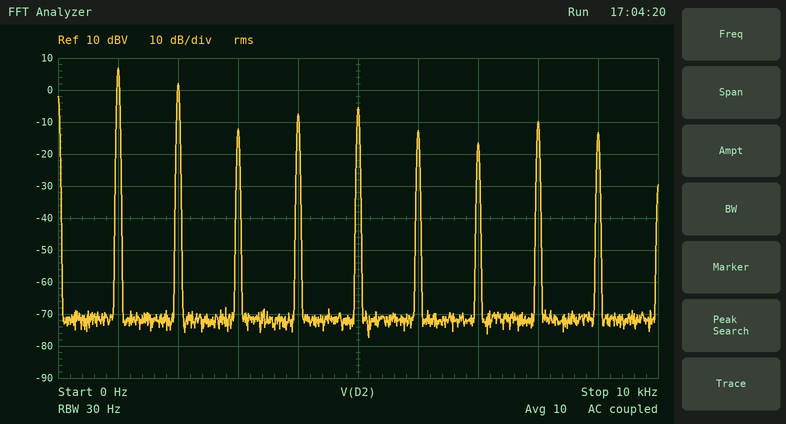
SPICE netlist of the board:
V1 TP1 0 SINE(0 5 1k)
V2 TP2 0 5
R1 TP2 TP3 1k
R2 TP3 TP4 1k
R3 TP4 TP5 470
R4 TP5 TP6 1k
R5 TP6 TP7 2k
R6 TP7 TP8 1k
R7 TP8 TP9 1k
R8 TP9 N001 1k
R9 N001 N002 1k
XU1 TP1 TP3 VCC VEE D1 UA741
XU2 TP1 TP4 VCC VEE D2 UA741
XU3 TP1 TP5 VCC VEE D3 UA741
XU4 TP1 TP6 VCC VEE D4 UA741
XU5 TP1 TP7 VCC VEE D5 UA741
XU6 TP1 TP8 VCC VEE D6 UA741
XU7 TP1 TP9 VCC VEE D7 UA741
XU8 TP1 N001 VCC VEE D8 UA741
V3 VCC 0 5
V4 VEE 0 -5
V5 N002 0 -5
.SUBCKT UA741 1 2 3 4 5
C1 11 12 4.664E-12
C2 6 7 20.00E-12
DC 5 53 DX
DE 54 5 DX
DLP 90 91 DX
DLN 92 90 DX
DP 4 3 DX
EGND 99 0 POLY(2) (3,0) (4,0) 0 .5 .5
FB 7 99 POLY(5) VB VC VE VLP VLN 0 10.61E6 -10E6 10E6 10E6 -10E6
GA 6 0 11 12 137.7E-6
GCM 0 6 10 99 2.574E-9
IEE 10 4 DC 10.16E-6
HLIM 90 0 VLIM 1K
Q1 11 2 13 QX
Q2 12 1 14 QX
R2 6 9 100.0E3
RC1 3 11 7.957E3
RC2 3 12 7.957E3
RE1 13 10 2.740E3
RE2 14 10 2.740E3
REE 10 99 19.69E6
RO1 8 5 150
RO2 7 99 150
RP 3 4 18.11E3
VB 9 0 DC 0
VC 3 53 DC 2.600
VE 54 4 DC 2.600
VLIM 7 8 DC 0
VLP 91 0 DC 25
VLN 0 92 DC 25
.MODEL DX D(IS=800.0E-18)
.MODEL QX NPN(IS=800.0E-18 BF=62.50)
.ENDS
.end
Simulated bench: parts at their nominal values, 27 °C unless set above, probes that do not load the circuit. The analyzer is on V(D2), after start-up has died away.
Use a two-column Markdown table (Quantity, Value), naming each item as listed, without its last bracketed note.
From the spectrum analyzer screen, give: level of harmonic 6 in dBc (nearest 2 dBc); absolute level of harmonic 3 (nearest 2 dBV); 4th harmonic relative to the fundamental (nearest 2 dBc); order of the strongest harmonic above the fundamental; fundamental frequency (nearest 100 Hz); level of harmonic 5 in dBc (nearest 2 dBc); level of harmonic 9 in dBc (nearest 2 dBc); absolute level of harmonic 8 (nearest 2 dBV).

| Quantity | Value |
|---|---|
| level of harmonic 6 in dBc | -20 dBc |
| absolute level of harmonic 3 | -12 dBV |
| 4th harmonic relative to the fundamental | -14 dBc |
| order of the strongest harmonic above the fundamental | 2 |
| fundamental frequency | 1.0 kHz |
| level of harmonic 5 in dBc | -12 dBc |
| level of harmonic 9 in dBc | -20 dBc |
| absolute level of harmonic 8 | -10 dBV |
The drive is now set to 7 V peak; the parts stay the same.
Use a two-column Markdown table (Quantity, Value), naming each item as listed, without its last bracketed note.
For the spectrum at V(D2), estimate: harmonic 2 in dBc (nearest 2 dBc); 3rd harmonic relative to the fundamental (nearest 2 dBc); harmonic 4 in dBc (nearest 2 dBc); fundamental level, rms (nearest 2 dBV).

| Quantity | Value |
|---|---|
| harmonic 2 in dBc | -8 dBc |
| 3rd harmonic relative to the fundamental | 2 dBc |
| harmonic 4 in dBc | 2 dBc |
| fundamental level, rms | -2 dBV |
